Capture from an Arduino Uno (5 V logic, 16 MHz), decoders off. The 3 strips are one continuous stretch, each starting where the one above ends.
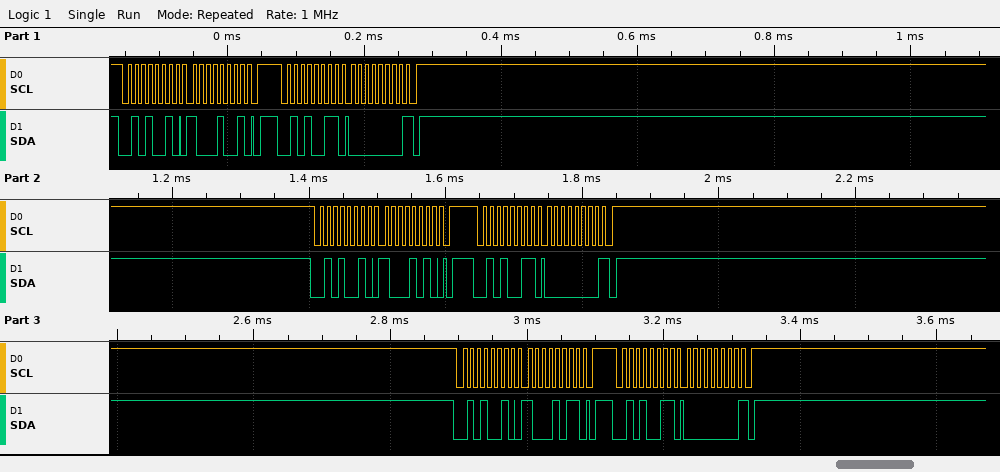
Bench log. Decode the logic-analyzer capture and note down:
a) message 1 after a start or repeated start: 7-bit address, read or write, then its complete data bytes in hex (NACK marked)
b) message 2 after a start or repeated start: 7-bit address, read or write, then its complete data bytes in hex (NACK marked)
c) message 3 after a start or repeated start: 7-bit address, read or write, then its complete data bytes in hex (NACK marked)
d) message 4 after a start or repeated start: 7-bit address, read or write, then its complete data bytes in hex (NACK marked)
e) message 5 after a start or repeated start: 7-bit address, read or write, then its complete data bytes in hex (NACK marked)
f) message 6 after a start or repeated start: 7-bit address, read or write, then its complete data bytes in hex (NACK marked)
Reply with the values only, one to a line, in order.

0x29 write: 89
0x29 read: 00 NACK
0x29 write: 8A
0x29 read: 00 NACK
0x29 write: 8B
0x29 read: 00 NACK
